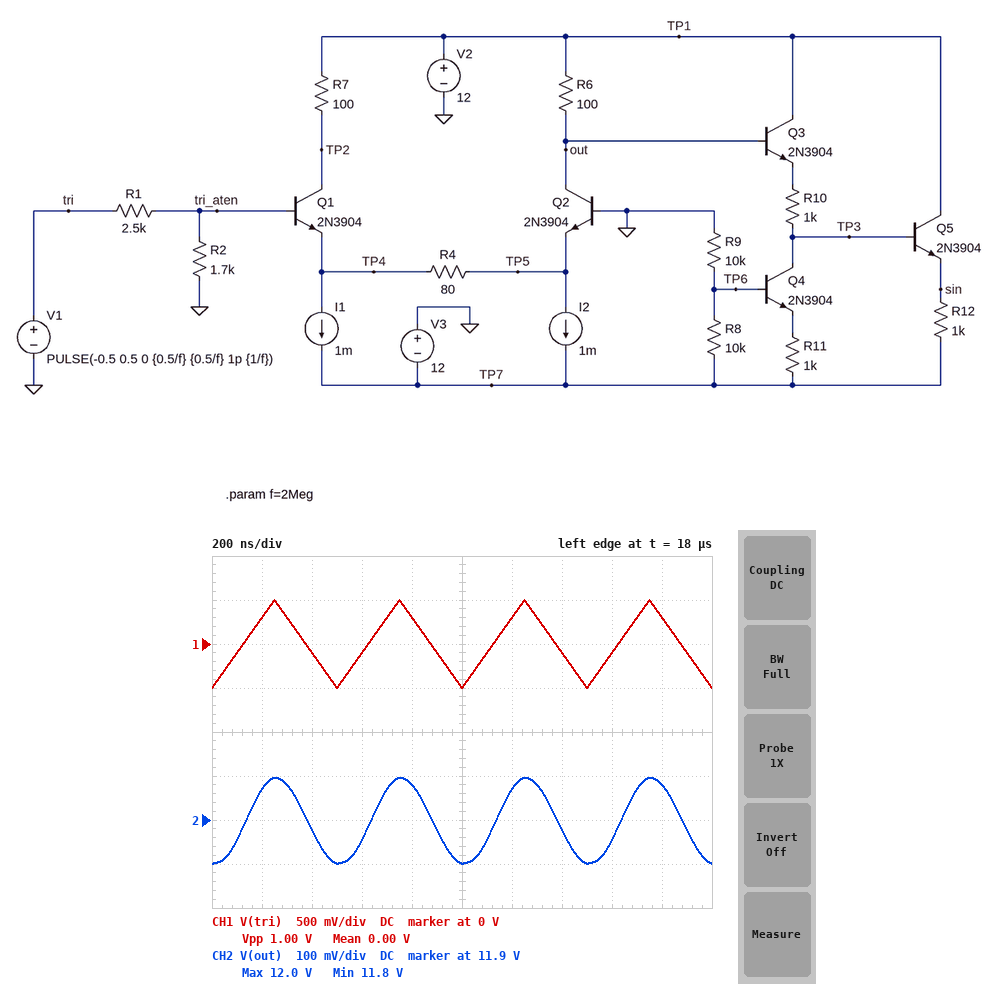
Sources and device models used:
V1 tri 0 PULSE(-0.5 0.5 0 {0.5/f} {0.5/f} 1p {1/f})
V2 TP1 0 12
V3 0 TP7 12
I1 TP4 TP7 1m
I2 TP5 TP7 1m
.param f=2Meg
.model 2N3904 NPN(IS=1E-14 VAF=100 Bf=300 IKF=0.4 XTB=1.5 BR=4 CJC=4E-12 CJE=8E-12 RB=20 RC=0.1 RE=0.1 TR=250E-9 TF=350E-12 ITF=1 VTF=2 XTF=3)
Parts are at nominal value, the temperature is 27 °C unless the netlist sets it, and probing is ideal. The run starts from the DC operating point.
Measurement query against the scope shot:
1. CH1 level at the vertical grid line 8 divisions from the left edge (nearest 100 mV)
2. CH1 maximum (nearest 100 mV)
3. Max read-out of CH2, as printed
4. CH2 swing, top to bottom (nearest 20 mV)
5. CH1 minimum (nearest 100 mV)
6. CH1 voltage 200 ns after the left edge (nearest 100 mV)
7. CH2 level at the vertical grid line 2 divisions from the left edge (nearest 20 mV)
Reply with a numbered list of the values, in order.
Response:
1. -100 mV
2. 500 mV
3. 12.0 V
4. 200 mV
5. -500 mV
6. 300 mV
7. 11.88 V
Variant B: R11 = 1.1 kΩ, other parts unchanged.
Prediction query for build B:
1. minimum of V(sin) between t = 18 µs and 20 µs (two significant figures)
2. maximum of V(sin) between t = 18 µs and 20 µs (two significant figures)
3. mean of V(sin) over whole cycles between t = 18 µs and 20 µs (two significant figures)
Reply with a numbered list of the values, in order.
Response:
1. 5.6 V
2. 5.8 V
3. 5.7 V
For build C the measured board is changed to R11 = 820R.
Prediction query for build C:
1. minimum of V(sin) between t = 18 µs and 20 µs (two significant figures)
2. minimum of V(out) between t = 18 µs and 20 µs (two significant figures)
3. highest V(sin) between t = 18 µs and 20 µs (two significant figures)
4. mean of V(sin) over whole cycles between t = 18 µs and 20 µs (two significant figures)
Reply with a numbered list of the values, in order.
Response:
1. 4.0 V
2. 12 V
3. 4.2 V
4. 4.1 V
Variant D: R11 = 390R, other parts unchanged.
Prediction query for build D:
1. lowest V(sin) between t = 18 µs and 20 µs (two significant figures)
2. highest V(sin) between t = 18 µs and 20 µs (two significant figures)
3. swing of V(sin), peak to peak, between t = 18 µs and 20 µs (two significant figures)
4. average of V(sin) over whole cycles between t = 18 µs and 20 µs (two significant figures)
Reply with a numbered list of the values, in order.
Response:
1. -2.6 V
2. -2.4 V
3. 170 mV
4. -2.5 V
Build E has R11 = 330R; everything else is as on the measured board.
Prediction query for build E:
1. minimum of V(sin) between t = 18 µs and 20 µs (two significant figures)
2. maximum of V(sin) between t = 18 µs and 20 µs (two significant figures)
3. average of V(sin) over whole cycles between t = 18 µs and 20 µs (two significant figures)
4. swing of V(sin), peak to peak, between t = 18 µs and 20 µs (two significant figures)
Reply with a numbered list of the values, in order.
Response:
1. -4.8 V
2. -4.6 V
3. -4.7 V
4. 160 mV
